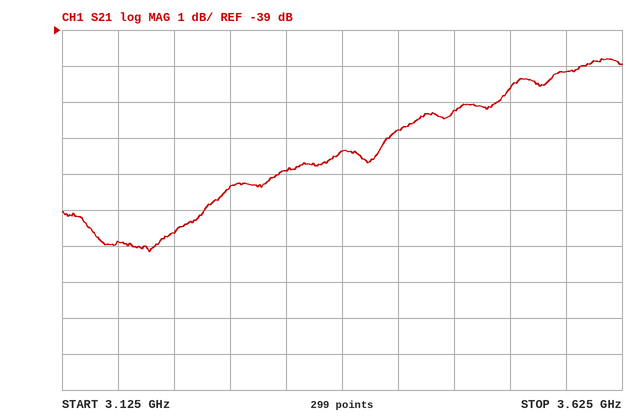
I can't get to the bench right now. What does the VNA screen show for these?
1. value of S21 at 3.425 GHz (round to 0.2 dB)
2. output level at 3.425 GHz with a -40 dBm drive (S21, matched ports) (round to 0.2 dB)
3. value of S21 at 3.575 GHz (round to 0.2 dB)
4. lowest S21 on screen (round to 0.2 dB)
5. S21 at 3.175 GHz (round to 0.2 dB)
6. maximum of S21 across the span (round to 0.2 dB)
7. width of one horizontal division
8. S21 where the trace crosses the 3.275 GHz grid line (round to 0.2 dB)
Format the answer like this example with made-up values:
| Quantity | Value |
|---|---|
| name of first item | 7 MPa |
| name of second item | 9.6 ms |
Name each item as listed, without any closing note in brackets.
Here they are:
| Quantity | Value |
|---|---|
| value of S21 at 3.425 GHz | -41.8 dB |
| output level at 3.425 GHz with a -40 dBm drive (S21, matched ports) | -81.8 dBm |
| value of S21 at 3.575 GHz | -40.2 dB |
| lowest S21 on screen | -45.2 dB |
| S21 at 3.175 GHz | -44.8 dB |
| maximum of S21 across the span | -39.8 dB |
| width of one horizontal division | 50 MHz |
| S21 where the trace crosses the 3.275 GHz grid line | -43.4 dB |
